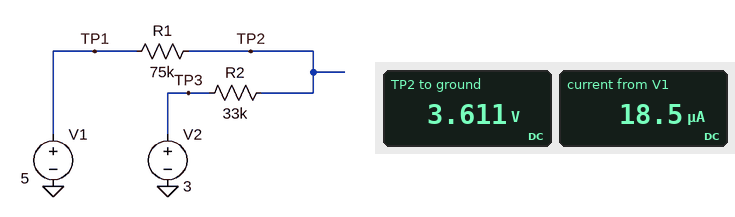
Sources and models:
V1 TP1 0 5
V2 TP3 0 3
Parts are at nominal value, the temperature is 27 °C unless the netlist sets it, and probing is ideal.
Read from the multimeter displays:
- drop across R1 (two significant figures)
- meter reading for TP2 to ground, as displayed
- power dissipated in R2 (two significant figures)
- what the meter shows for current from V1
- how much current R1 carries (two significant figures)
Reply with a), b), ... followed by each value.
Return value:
a) 1.4 V
b) 3.611 V
c) 11 µW
d) 18.5 µA
e) 19 µA
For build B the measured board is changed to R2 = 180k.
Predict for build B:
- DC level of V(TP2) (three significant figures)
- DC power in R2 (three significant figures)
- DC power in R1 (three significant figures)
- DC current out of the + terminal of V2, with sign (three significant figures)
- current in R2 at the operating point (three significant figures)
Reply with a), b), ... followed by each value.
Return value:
a) 4.41 V
b) 11.1 µW
c) 4.61 µW
d) -7.84 µA
e) 7.84 µA
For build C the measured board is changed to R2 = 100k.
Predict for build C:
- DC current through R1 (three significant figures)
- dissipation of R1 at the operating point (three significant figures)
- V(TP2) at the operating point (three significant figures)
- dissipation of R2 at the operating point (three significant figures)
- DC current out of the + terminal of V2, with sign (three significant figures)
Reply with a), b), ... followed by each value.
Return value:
a) 11.4 µA
b) 9.80 µW
c) 4.14 V
d) 13.1 µW
e) -11.4 µA
